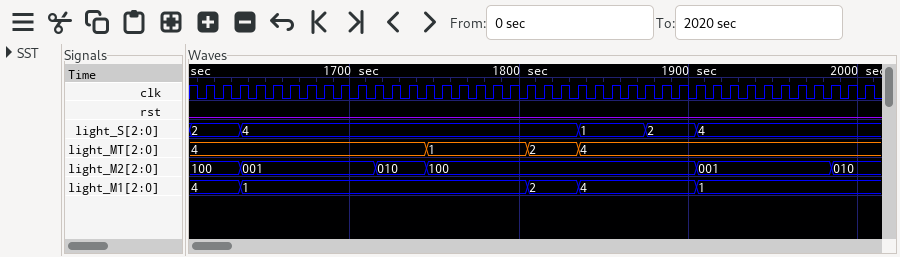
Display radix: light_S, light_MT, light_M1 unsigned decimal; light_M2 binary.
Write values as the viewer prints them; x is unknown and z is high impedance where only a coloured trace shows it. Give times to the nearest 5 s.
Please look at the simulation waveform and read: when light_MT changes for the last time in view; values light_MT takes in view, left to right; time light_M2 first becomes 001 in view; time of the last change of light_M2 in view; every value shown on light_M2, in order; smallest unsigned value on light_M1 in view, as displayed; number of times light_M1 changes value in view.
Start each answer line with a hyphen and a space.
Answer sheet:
- 1835 s
- 4, 1, 2, 4
- 1635 s
- 1985 s
- 100, 001, 010, 100, 001, 010
- 1
- 4
